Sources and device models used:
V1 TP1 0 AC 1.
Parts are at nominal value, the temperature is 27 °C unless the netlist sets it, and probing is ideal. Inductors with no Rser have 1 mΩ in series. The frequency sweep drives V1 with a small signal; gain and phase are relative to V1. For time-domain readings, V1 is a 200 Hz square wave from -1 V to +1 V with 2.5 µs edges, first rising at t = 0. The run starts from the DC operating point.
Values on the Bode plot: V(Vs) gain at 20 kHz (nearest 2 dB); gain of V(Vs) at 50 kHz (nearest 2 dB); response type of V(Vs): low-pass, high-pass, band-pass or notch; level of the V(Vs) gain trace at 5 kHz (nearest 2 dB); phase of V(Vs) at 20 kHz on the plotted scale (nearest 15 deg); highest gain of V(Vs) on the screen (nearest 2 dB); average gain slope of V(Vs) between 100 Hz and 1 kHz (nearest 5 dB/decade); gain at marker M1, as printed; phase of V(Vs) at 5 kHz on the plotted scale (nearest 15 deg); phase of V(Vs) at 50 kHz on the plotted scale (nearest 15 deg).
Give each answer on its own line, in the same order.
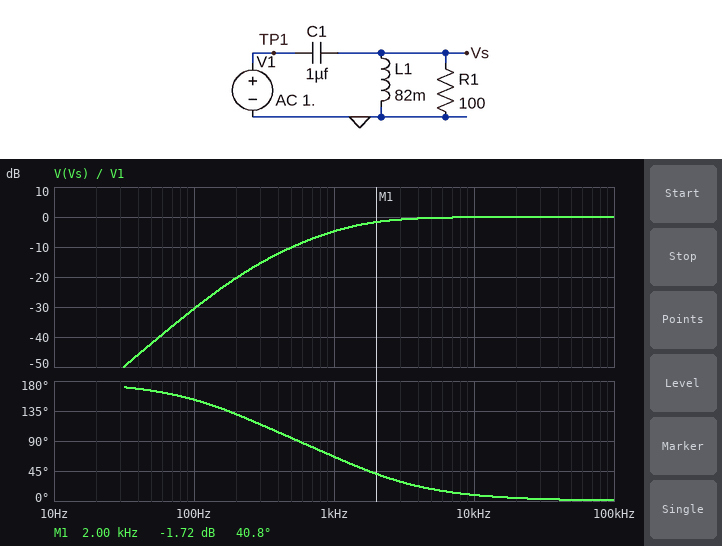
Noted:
0 dB
0 dB
high-pass
0 dB
0 deg
0 dB
25 dB/decade
-1.72 dB
15 deg
0 deg
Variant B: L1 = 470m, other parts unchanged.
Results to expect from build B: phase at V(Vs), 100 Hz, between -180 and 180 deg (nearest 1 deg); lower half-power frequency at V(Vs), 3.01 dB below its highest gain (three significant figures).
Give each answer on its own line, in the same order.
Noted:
105 deg
1.56 kHz
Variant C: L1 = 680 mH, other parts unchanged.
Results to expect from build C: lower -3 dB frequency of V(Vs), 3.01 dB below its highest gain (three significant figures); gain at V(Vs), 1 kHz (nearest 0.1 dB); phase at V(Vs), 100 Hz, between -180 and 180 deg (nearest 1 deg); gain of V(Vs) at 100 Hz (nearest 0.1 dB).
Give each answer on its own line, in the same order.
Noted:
1.57 kHz
-5.4 dB
100 deg
-24.2 dB
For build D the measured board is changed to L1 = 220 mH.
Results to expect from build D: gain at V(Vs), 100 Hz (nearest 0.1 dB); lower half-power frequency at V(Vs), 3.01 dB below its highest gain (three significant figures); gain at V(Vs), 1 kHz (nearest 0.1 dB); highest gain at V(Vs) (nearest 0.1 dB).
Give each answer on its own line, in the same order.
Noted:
-25.6 dB
1.52 kHz
-5.2 dB
0 dB
